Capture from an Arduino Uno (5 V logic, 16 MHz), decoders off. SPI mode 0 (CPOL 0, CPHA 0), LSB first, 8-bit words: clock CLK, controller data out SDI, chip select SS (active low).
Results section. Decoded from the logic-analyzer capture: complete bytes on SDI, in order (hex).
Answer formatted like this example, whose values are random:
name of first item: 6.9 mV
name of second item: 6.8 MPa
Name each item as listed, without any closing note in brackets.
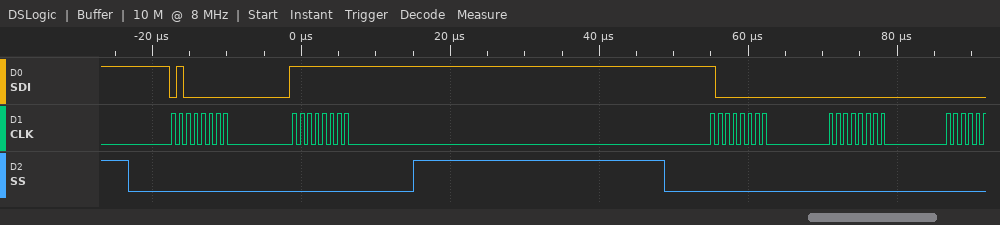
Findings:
complete bytes on SDI, in order: 02 FF 01 00
